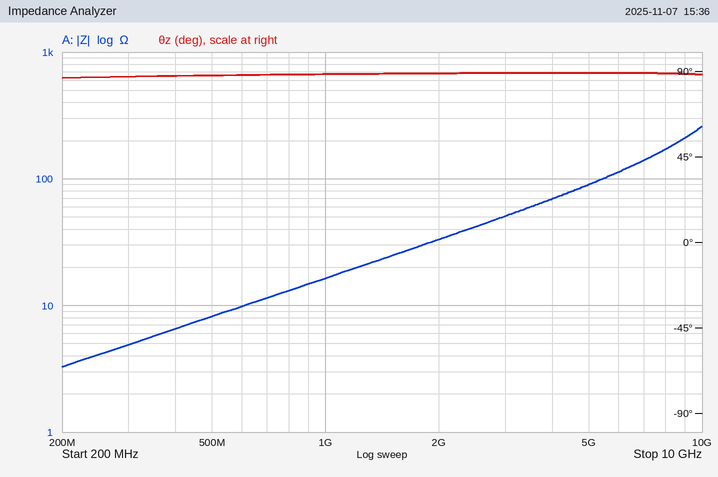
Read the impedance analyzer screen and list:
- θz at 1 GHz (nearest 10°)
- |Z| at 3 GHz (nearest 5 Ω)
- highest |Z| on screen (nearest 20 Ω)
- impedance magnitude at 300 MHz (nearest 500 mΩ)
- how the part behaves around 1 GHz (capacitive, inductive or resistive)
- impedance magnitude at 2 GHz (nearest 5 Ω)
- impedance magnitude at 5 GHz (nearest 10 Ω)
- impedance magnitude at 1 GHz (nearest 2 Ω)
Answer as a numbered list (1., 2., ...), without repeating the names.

1. 90°
2. 50 Ω
3. 260 Ω
4. 5.0 Ω
5. inductive
6. 35 Ω
7. 90 Ω
8. 16 Ω
